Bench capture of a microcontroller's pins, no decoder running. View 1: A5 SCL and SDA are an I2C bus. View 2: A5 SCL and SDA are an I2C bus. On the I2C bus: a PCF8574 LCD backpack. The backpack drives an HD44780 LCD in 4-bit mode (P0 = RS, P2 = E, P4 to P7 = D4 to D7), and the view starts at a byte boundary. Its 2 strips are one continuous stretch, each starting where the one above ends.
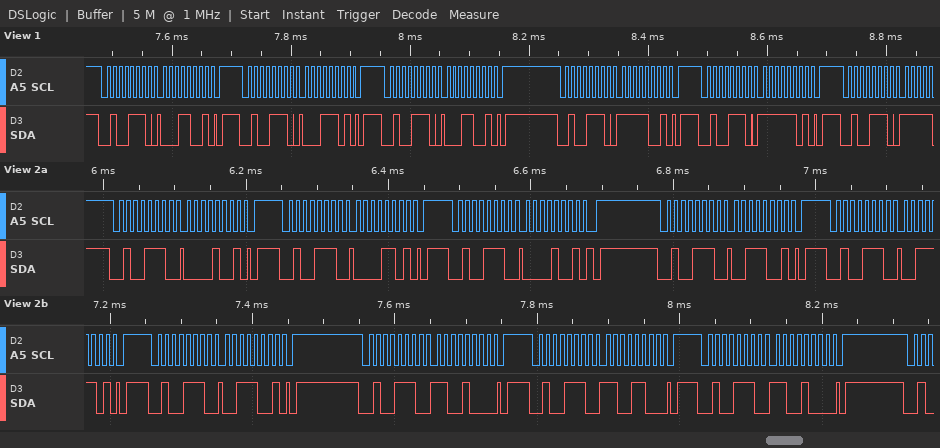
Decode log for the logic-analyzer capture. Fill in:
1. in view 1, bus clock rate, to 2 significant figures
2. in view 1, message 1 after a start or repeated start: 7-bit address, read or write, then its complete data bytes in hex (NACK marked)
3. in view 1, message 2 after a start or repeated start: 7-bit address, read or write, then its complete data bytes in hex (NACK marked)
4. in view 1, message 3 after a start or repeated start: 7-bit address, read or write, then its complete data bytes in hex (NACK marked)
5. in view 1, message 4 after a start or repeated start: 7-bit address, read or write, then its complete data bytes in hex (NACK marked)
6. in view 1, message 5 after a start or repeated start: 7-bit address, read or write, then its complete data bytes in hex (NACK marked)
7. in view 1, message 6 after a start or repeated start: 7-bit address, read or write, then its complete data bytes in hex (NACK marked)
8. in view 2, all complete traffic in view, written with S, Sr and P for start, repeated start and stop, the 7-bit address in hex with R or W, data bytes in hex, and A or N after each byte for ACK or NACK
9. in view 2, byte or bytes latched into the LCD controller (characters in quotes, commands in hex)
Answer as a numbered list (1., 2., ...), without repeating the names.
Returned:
1. 100 kHz
2. 0x27 write: 19
3. 0x27 write: 1D
4. 0x27 write: 19
5. 0x27 write: F9
6. 0x27 write: FD
7. 0x27 write
8. S 27W A 09 A P S 27W A 0D A P S 27W A 09 A P S 27W A 39 A P S 27W A 3D A P S 27W A 39 A P S 27W A C8 A P S 27W A CC A P S 27W A C8 A P
9. data 0x03
